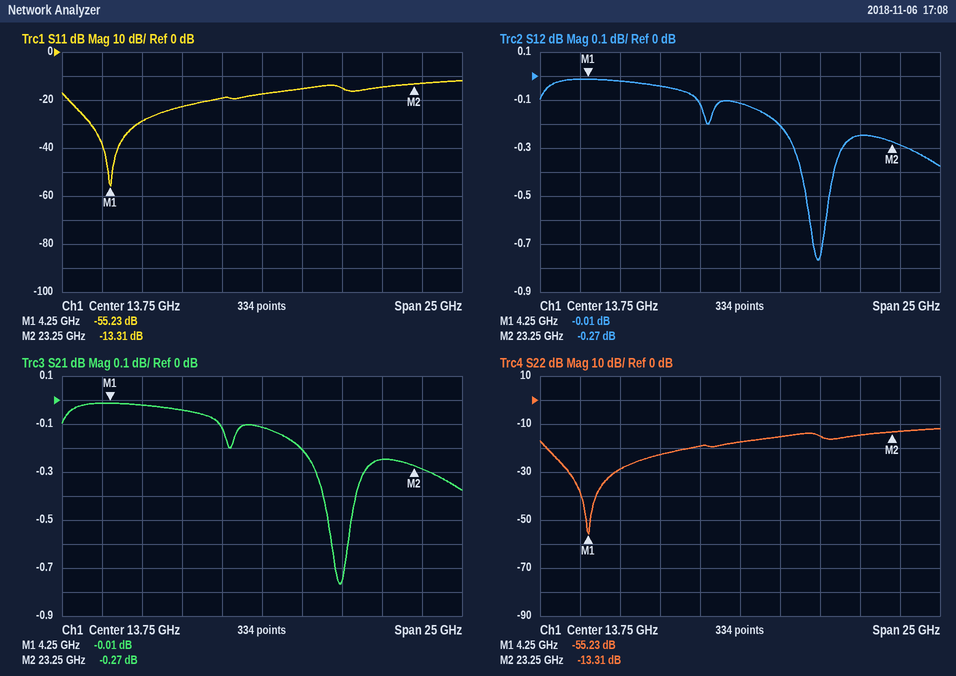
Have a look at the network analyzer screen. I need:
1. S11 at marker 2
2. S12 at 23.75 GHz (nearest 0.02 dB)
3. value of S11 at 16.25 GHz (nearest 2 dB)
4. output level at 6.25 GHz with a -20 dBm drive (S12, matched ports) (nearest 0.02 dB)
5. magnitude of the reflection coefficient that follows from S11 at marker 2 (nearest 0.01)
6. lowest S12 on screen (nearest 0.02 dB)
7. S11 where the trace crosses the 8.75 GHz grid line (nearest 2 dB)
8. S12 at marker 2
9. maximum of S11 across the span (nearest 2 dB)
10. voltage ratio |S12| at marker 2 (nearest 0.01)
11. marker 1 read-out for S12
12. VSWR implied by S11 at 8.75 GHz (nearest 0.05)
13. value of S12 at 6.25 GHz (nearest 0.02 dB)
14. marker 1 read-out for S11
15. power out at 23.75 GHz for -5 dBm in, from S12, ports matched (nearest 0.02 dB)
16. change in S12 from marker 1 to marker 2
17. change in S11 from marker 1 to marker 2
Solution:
-13.31 dB
-0.28 dB
-16 dB
-20.02 dBm
0.22
-0.76 dB
-22 dB
-0.27 dB
-12 dB
0.97
-0.01 dB
1.15
-0.02 dB
-55.23 dB
-5.28 dBm
-0.26 dB
41.92 dB
